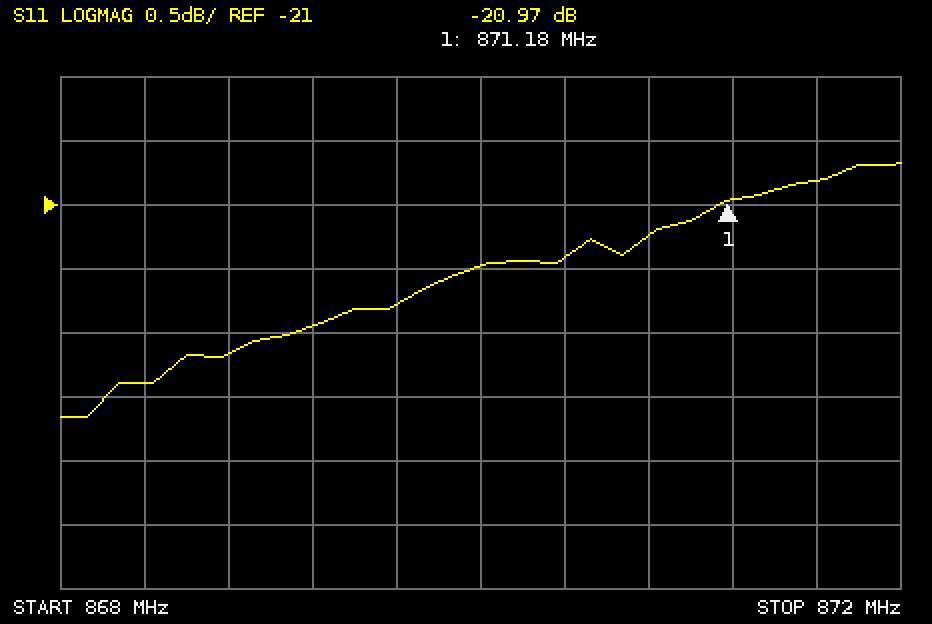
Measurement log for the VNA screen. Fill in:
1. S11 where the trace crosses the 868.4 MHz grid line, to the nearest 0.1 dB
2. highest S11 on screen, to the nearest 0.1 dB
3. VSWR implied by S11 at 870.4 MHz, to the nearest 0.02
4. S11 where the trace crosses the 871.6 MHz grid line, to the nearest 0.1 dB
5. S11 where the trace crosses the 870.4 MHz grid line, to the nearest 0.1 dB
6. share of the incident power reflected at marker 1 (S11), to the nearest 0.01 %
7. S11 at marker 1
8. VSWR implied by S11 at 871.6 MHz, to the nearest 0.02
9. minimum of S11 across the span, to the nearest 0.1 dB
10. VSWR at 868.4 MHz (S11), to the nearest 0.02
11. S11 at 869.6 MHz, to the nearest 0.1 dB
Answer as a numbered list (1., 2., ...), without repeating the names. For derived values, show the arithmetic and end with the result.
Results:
1. -22.4 dB
2. -20.7 dB
3. |Γ| = 10^(-21.4/20) = 0.0851; VSWR = (1 + 0.0851)/(1 − 0.0851) ≈ 1.19, so 1.18 to the nearest 0.02
4. -20.8 dB
5. -21.4 dB
6. 10^(-20.97/10) ≈ 0.80 %
7. -20.97 dB
8. |Γ| = 10^(-20.8/20) = 0.0912; VSWR = (1 + 0.0912)/(1 − 0.0912) ≈ 1.20
9. -22.7 dB
10. |Γ| = 10^(-22.4/20) = 0.0759; VSWR = (1 + 0.0759)/(1 − 0.0759) ≈ 1.16
11. -21.8 dB
